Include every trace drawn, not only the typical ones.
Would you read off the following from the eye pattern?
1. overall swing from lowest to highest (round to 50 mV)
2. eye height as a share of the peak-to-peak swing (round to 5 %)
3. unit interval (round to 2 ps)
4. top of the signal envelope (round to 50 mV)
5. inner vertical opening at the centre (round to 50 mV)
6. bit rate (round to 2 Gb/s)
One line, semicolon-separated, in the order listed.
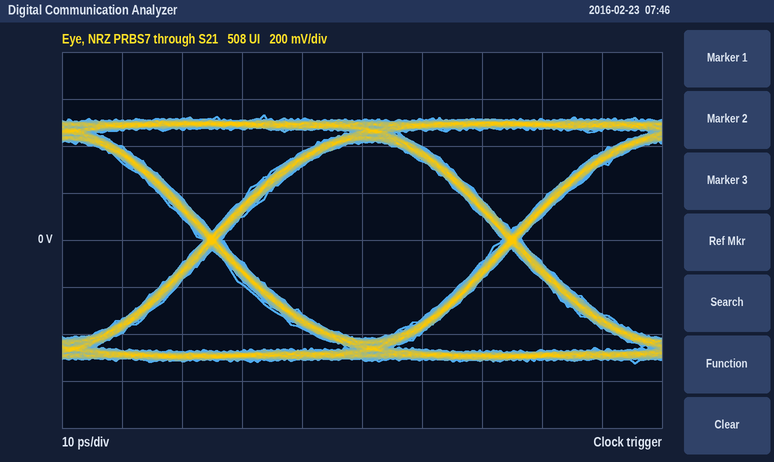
1.05 V; 80 %; 50 ps; 550 mV; 850 mV; 20 Gb/s
